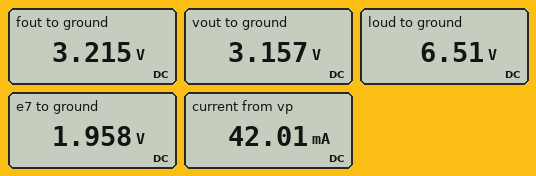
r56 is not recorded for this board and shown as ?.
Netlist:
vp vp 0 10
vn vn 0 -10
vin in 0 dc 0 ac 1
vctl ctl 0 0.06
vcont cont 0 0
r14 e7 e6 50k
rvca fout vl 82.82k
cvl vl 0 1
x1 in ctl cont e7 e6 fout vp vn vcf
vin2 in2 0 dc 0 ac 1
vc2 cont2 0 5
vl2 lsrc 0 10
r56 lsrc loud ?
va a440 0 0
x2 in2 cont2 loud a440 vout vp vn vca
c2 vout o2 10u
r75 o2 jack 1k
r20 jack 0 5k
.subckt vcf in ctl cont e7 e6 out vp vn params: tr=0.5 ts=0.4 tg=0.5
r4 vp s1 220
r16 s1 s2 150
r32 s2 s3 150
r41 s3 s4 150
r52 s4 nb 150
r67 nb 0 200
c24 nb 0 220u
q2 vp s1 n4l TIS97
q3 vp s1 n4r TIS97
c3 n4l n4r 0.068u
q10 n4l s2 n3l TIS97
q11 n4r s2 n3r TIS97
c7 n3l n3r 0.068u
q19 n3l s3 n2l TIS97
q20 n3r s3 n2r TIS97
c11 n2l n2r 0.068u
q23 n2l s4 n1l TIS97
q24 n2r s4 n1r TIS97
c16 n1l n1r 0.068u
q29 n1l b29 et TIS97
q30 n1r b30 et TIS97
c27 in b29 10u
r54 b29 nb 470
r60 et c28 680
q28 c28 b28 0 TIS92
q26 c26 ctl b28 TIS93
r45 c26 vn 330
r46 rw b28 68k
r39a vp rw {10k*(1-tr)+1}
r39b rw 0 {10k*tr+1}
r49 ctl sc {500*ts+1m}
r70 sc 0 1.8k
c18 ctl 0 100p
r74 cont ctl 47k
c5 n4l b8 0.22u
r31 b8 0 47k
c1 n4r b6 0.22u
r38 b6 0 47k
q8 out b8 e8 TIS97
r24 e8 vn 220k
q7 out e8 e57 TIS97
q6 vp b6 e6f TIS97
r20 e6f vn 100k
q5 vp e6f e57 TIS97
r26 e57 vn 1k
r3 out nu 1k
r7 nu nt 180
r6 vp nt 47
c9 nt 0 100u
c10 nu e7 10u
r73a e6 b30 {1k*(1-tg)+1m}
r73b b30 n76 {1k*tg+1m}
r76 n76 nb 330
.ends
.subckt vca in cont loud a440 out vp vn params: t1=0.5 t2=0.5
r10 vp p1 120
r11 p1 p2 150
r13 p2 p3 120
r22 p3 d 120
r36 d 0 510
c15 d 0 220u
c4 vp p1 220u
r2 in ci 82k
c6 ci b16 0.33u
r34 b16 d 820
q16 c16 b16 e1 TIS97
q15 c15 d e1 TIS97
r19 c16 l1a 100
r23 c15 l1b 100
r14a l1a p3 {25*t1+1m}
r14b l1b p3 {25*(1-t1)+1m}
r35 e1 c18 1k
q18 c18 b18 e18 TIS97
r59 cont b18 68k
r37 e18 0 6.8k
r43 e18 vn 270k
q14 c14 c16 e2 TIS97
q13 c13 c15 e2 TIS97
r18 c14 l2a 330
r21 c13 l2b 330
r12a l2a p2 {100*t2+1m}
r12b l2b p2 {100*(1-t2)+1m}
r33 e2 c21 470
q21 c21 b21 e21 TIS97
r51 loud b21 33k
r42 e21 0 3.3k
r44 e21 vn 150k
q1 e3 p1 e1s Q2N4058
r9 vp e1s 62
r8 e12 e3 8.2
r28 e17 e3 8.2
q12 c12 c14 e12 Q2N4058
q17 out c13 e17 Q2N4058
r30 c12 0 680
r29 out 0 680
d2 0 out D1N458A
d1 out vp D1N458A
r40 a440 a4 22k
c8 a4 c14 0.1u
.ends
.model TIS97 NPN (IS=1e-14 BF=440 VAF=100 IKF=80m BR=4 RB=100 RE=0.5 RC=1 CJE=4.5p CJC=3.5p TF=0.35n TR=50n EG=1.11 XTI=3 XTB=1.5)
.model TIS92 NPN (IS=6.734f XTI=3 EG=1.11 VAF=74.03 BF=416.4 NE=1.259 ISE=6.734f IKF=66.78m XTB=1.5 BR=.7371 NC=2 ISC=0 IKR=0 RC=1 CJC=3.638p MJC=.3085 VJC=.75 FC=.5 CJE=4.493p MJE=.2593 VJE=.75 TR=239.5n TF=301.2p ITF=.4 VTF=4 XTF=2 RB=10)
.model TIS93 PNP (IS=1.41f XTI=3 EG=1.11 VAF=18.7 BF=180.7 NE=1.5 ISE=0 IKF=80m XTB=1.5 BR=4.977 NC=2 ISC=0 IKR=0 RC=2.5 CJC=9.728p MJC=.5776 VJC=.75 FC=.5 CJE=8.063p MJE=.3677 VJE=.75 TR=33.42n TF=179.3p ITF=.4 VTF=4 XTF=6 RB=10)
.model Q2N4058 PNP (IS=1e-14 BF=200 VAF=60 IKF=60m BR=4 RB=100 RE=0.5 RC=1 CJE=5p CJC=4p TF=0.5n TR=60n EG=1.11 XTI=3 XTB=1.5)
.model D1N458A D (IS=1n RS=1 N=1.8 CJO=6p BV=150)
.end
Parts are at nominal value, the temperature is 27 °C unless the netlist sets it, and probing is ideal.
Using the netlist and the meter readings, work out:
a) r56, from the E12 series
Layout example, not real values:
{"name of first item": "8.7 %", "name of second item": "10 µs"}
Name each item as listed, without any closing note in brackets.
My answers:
{"r56, from the E12 series": "82 kΩ"}
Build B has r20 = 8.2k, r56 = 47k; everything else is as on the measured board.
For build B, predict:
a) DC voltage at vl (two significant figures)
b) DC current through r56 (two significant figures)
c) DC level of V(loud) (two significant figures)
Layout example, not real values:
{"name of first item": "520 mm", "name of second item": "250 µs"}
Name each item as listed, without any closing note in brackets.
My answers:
{"DC voltage at vl": "3.2 V", "DC current through r56": "61 µA", "DC level of V(loud)": "7.1 V"}
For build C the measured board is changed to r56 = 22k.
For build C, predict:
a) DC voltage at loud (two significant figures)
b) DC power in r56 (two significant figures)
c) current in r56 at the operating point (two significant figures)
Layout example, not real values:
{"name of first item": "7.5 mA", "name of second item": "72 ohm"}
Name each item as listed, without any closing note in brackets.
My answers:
{"DC voltage at loud": "8.1 V", "DC power in r56": "170 µW", "current in r56 at the operating point": "88 µA"}
